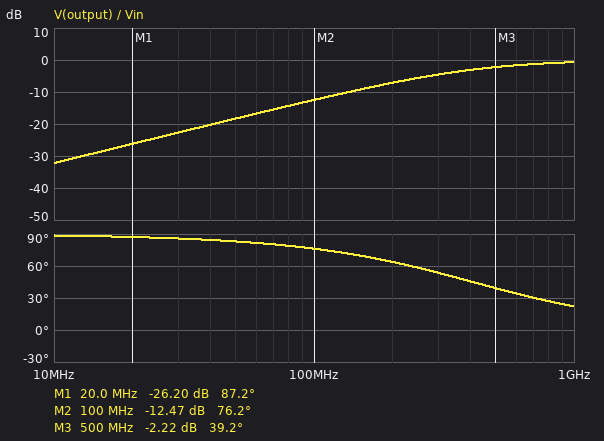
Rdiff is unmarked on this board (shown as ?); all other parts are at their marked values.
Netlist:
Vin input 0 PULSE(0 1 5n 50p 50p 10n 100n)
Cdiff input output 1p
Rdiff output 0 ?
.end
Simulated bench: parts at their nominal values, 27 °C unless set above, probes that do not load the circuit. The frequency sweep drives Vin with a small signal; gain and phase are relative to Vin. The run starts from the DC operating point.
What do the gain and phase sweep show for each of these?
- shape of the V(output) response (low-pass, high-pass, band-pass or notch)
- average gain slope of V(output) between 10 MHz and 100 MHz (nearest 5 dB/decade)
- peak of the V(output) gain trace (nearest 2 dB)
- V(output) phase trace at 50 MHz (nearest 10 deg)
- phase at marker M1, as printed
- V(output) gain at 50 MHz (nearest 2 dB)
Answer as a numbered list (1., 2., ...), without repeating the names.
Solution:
1. high-pass
2. 20 dB/decade
3. 0 dB
4. 80 deg
5. 87.2 deg
6. -18 dB
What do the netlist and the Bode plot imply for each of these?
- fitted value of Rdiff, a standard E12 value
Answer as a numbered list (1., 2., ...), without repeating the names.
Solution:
1. 390 Ω
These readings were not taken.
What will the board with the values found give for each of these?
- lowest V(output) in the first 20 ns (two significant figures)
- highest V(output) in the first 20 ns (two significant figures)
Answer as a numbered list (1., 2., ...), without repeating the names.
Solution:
1. -940 mV
2. 940 mV
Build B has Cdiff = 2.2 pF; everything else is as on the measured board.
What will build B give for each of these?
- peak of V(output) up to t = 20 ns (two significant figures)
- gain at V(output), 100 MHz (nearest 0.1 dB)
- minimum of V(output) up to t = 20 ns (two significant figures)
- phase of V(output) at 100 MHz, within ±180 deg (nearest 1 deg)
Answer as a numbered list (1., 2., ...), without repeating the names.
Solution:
1. 970 mV
2. -6.5 dB
3. -970 mV
4. 62 deg
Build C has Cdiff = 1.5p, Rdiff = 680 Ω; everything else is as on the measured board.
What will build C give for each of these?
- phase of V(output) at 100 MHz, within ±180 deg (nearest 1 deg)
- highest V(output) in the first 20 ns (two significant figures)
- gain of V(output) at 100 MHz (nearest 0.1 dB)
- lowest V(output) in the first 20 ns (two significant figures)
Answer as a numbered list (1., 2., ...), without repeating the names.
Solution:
1. 57 deg
2. 980 mV
3. -5.4 dB
4. -980 mV
